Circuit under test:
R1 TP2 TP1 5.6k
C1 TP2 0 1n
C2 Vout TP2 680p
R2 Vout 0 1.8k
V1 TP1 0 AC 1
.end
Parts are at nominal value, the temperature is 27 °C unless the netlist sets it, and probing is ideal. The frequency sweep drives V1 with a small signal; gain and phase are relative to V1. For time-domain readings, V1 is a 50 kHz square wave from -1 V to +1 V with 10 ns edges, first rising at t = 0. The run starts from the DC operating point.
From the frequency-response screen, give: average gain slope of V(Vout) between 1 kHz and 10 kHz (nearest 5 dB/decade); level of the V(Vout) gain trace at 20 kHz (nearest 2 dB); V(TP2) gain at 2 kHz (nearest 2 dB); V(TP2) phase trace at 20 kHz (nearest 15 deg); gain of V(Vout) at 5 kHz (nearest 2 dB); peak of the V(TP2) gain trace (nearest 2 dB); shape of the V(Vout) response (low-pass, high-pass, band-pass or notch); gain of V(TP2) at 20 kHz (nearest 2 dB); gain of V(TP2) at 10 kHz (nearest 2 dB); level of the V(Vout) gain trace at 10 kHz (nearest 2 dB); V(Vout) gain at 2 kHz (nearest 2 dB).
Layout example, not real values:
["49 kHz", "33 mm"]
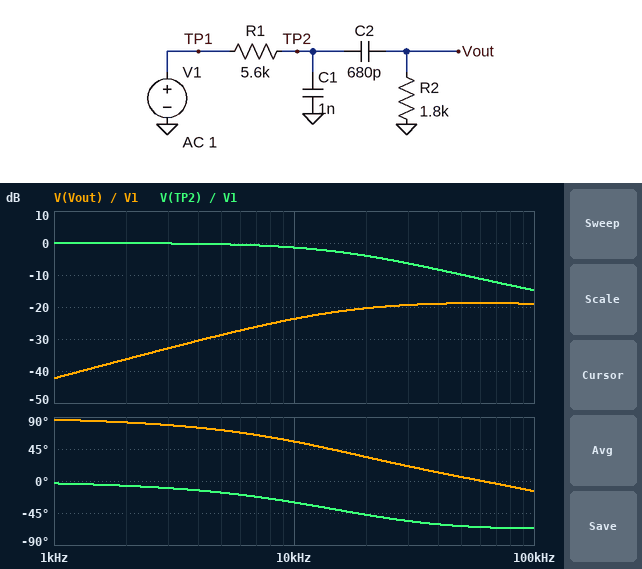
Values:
["20 dB/decade", "-20 dB", "0 dB", "-45 deg", "-28 dB", "0 dB", "high-pass", "-4 dB", "-2 dB", "-24 dB", "-36 dB"]
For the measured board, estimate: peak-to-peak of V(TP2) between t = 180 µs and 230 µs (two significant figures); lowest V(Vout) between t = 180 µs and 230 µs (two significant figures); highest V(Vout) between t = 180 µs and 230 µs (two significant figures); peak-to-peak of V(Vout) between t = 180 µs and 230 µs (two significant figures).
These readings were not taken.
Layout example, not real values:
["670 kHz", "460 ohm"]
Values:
["990 mV", "-140 mV", "140 mV", "290 mV"]
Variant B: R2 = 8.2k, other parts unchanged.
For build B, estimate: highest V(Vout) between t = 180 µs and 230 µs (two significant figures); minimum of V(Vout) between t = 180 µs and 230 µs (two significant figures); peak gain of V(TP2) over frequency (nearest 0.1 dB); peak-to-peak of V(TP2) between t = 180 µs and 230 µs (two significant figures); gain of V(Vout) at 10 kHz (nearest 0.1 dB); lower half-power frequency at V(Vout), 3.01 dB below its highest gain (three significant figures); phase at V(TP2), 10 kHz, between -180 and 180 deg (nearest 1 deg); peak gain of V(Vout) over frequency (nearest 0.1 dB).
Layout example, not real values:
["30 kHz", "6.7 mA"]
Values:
["380 mV", "-380 mV", "0 dB", "1.1 V", "-11.3 dB", "9.45 kHz", "-28 deg", "-8.6 dB"]
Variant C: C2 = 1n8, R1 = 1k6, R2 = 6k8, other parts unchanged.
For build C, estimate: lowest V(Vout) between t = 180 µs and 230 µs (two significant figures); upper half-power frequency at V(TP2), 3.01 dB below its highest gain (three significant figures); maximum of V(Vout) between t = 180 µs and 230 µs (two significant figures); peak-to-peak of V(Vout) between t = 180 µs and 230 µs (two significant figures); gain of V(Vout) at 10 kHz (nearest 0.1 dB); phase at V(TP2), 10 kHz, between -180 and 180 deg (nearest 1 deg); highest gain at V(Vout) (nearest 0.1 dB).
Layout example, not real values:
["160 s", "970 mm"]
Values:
["-800 mV", "65.6 kHz", "800 mV", "1.6 V", "-5.2 dB", "-11 deg", "-2.7 dB"]
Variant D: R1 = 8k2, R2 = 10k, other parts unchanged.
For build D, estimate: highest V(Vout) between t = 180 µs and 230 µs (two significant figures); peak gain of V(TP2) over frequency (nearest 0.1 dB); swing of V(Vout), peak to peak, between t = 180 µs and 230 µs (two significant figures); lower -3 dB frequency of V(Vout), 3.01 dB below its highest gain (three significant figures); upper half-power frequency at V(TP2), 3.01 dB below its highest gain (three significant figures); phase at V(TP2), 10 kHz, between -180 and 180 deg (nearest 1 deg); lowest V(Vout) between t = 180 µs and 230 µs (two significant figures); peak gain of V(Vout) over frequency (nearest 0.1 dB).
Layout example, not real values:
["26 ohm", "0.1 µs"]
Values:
["310 mV", "0 dB", "620 mV", "6.92 kHz", "10.4 kHz", "-36 deg", "-310 mV", "-9.6 dB"]
